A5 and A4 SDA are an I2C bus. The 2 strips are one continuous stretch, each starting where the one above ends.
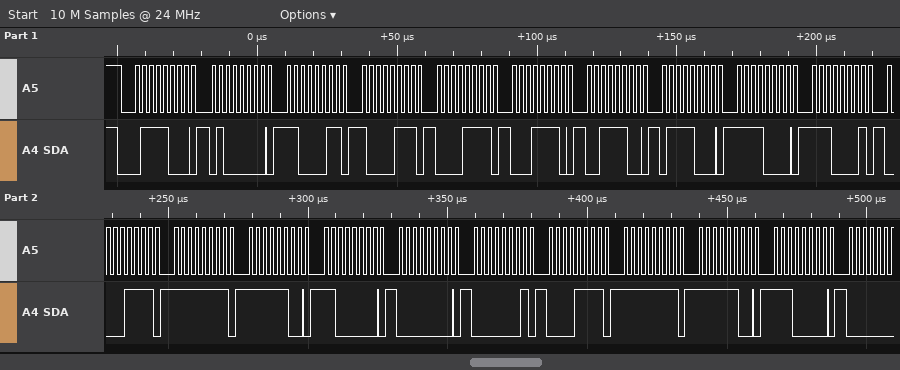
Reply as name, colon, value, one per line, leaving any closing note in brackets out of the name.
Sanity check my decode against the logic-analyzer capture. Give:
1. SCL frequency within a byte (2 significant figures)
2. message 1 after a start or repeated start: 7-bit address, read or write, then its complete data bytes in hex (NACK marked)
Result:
SCL frequency within a byte: 400 kHz
message 1 after a start or repeated start: 7-bit address, read or write, then its complete data bytes in hex: 0x3C write: 40 C3 87 0F 1E 3C 78 F0 E1 0F FF FC C0 00 01 0F FF FC E0
